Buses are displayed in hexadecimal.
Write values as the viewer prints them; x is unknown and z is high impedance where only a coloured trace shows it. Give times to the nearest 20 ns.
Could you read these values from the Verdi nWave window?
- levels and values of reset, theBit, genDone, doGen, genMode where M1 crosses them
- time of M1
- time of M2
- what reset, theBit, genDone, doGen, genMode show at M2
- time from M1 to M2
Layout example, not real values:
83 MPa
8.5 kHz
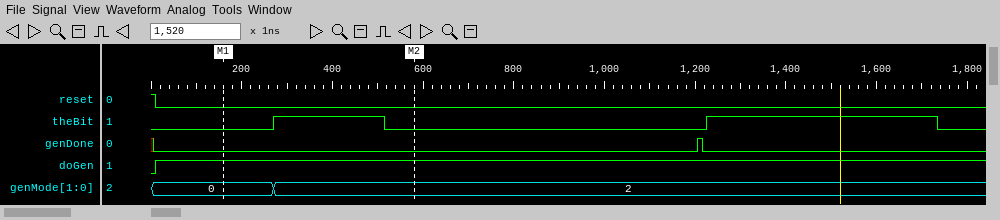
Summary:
reset=0, theBit=0, genDone=0, doGen=1, genMode=0
160 ns
580 ns
reset=0, theBit=0, genDone=0, doGen=1, genMode=2
420 ns
